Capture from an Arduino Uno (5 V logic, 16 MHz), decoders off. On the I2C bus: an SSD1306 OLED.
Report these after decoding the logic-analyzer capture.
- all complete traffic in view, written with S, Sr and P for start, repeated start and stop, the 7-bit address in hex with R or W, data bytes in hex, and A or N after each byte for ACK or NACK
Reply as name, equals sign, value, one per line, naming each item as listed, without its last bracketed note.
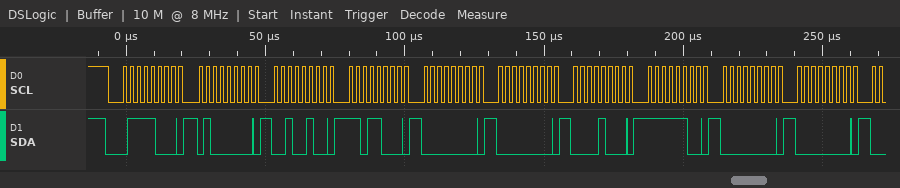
all complete traffic in view, written with S, Sr and P for start, repeated start and stop, the 7-bit address in hex with R or W, data bytes in hex, and A or N after each byte for ACK or NACK = S 3CW A 40 A 24 A D8 A 00 A 00 A 08 A FC A 00 A 00 A
